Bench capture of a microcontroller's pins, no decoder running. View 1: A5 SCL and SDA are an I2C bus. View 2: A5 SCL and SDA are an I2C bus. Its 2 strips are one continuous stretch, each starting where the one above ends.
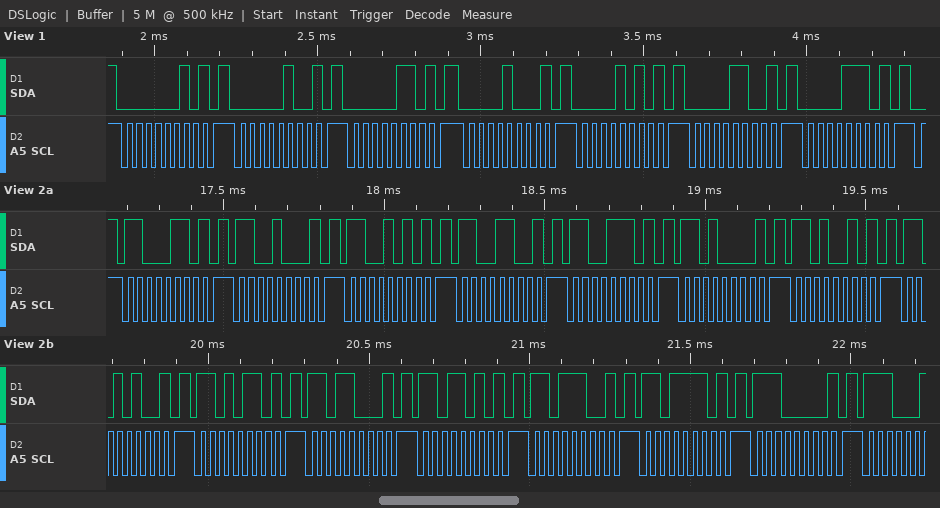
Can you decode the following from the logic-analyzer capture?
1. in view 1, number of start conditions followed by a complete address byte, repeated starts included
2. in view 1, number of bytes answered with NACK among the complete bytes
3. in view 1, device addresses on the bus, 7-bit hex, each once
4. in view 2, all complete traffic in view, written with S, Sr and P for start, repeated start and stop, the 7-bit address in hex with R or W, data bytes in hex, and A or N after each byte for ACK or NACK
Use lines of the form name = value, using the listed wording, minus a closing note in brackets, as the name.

in view 1, number of start conditions followed by a complete address byte, repeated starts included = 7
in view 1, number of bytes answered with NACK among the complete bytes = 7
in view 1, device addresses on the bus, 7-bit hex, each once = 0x01 0x02 0x03 0x04 0x05 0x06 0x07
in view 2, all complete traffic in view, written with S, Sr and P for start, repeated start and stop, the 7-bit address in hex with R or W, data bytes in hex, and A or N after each byte for ACK or NACK = S 63W N P S 64W N P S 65W N P S 66W N P S 67W N P S 68W N P S 69W N P S 6AW N P S 6BW N P S 6CW N P S 6DW N P S 6EW N P S 6FW N P S 70W N P
